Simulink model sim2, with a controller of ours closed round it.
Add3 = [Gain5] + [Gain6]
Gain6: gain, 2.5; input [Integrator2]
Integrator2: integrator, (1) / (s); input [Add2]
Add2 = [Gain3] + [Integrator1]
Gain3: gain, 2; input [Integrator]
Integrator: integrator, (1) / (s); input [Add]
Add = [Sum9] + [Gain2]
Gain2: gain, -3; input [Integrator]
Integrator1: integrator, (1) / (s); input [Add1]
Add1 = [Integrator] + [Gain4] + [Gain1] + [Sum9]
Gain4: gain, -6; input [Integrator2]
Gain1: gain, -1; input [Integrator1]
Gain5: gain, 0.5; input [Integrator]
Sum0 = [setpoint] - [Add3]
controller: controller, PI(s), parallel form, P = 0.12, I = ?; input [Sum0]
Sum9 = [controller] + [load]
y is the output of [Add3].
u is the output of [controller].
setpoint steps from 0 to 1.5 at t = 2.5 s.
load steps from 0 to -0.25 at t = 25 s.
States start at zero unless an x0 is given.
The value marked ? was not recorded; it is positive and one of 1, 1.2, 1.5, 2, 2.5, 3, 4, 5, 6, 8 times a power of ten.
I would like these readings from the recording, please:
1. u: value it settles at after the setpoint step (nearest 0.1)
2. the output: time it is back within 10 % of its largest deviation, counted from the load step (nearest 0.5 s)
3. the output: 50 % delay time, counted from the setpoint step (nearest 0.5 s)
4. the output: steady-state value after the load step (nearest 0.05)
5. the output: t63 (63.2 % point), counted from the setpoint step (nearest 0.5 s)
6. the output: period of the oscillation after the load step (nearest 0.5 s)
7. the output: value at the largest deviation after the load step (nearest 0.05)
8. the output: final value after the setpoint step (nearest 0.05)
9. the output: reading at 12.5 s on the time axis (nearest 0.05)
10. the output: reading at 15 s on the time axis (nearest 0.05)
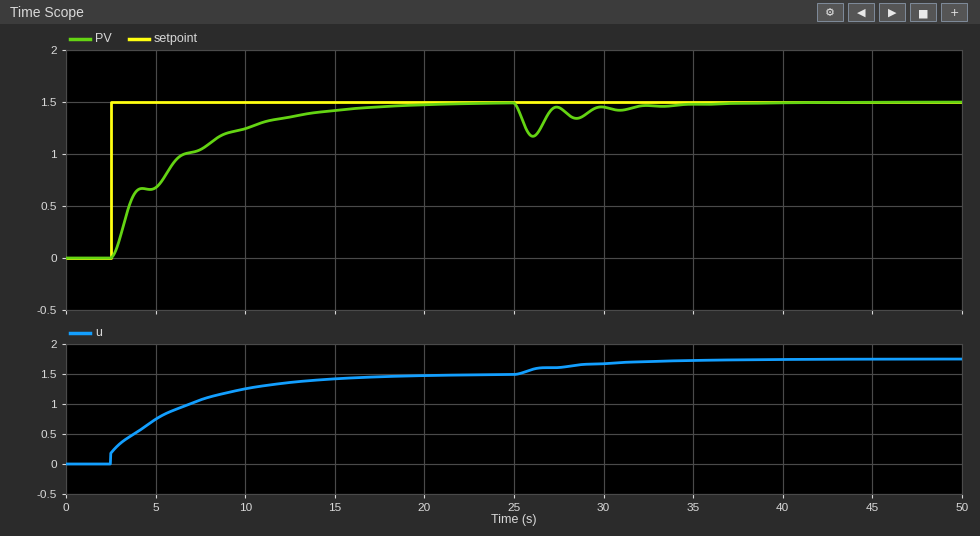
1.5
9.0 s
3.0 s
1.50
3.5 s
2.5 s
1.15
1.50
1.35
1.40
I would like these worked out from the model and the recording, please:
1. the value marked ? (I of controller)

0.25
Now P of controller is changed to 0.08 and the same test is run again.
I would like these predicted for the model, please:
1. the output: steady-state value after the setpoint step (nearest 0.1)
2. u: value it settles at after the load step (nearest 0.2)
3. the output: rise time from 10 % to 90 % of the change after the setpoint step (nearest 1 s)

1.5
1.8
9 s
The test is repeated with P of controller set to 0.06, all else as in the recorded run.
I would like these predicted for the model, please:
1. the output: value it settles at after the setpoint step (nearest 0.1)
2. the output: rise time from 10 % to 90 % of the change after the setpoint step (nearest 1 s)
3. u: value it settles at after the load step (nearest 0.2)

1.5
9 s
1.8
